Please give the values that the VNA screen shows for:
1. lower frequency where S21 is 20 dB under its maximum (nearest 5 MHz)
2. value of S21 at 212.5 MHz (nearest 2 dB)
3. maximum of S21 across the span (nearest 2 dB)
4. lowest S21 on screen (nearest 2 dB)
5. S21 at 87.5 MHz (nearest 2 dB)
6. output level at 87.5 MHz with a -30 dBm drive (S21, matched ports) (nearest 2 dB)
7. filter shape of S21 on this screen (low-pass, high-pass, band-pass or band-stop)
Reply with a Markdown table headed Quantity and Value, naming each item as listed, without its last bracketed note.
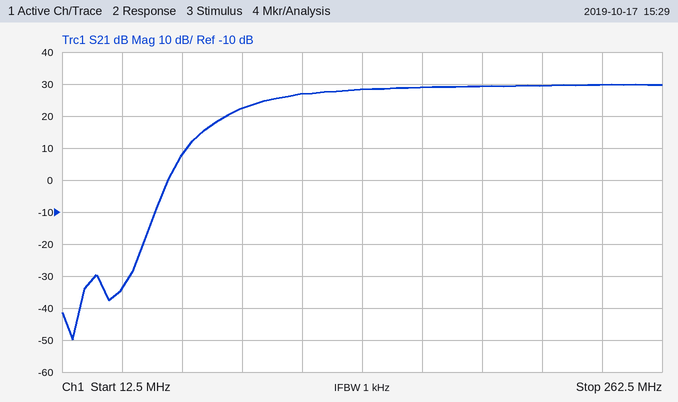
| Quantity | Value |
|---|---|
| lower frequency where S21 is 20 dB under its maximum | 65 MHz |
| value of S21 at 212.5 MHz | 30 dB |
| maximum of S21 across the span | 30 dB |
| lowest S21 on screen | -50 dB |
| S21 at 87.5 MHz | 22 dB |
| output level at 87.5 MHz with a -30 dBm drive (S21, matched ports) | -8 dBm |
| filter shape of S21 on this screen | high-pass |
